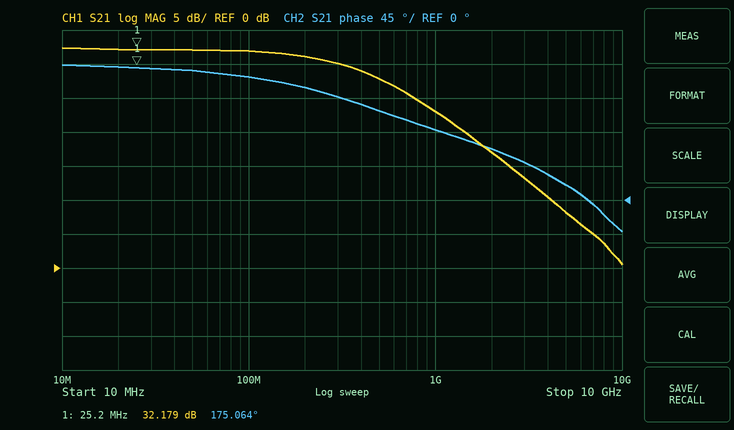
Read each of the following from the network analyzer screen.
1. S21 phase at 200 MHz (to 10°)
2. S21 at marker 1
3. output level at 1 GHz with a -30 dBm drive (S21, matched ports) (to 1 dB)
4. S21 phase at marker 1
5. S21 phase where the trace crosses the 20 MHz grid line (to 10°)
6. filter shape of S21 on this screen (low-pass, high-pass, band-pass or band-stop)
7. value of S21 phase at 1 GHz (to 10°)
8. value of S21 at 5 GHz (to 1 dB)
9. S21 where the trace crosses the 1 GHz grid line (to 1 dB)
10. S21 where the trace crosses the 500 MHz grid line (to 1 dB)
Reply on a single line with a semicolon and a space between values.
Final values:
150°; 32.179 dB; -7 dBm; 175.064°; 180°; low-pass; 90°; 8 dB; 23 dB; 28 dB
